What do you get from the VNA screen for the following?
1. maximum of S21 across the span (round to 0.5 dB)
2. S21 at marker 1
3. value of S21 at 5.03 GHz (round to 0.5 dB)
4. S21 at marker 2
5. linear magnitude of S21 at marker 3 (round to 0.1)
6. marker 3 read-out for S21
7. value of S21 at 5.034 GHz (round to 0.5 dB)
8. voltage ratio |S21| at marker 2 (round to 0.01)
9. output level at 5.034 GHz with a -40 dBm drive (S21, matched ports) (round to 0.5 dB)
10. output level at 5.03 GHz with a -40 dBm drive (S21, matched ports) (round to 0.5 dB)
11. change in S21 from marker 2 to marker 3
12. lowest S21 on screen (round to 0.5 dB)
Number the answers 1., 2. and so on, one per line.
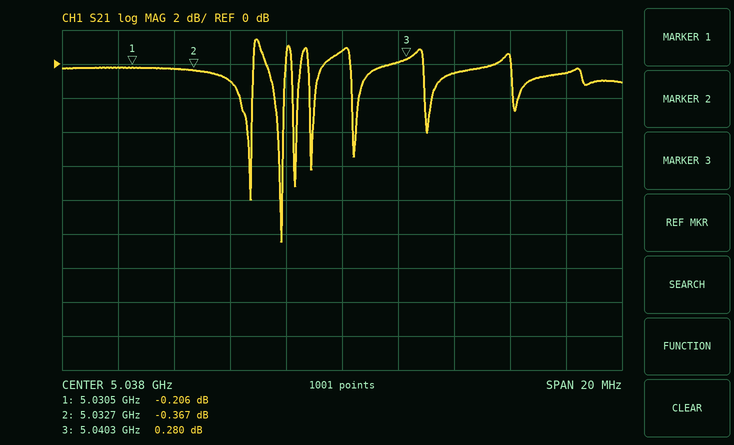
1. 1.5 dB
2. -0.206 dB
3. 0.0 dB
4. -0.367 dB
5. 1.0
6. 0.280 dB
7. -1.0 dB
8. 0.96
9. -41.0 dBm
10. -40.0 dBm
11. 0.647 dB
12. -10.5 dB
